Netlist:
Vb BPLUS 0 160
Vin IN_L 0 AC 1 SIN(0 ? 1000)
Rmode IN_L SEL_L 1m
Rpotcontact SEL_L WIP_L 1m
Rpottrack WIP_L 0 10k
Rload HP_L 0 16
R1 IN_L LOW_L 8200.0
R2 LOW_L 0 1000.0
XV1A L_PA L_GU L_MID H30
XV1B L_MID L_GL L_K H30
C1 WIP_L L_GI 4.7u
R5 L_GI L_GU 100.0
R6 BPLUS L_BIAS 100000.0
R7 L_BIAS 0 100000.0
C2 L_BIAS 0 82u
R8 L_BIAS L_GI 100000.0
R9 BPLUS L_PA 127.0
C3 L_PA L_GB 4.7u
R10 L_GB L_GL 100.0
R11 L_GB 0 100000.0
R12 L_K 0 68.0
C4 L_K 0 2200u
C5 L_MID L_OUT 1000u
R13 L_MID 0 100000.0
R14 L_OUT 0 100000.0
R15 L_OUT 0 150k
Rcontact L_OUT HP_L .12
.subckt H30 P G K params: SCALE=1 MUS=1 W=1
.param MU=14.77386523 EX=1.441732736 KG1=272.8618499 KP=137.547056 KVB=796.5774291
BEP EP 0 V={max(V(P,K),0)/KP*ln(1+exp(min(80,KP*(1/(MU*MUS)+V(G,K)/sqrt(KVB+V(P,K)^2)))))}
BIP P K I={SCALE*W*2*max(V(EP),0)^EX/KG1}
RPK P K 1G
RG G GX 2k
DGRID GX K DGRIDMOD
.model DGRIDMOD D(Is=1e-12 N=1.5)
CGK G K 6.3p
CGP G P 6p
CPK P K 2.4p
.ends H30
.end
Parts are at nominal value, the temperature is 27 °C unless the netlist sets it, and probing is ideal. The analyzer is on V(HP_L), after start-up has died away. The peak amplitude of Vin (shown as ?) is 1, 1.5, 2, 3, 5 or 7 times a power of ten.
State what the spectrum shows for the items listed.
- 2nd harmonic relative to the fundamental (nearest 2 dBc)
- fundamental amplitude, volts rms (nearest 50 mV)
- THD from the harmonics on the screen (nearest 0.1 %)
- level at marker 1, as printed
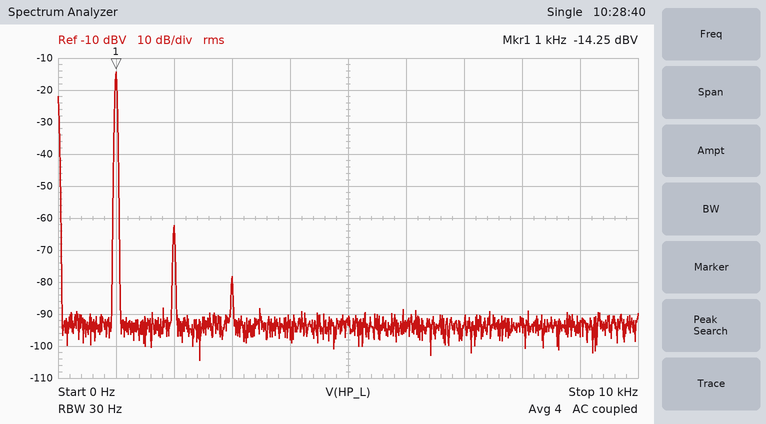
-48 dBc
200 mV
0.4 %
-14.25 dBV
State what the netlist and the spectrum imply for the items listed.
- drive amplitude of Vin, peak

700 mV
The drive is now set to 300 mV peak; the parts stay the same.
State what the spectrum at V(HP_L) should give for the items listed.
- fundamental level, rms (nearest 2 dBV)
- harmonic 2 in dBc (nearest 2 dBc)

-22 dBV
-56 dBc
